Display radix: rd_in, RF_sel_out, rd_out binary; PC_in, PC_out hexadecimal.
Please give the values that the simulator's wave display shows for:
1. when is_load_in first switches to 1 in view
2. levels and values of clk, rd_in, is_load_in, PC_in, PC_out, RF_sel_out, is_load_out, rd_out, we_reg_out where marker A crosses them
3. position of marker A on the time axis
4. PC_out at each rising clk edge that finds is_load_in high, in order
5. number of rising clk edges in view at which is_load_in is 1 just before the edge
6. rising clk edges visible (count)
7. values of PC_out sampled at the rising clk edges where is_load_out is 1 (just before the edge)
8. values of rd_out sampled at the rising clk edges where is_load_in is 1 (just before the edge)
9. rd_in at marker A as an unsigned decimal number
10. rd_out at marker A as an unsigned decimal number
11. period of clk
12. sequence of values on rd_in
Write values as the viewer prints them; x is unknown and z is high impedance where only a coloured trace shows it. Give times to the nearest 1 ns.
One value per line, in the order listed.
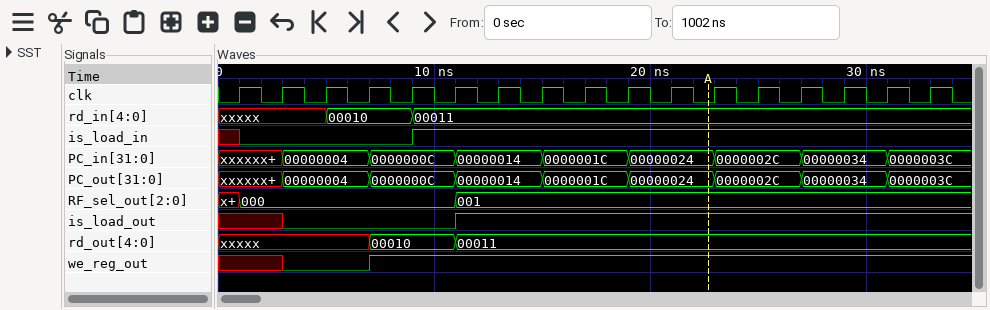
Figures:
9 ns
clk=0, rd_in=00011, is_load_in=1, PC_in=00000024, PC_out=00000024, RF_sel_out=001, is_load_out=1, rd_out=00011, we_reg_out=1
23 ns
0000000C, 00000014, 00000014, 0000001C, 0000001C, 00000024, 00000024, 0000002C, 0000002C, 00000034, 00000034, 0000003C
12
17
00000014, 00000014, 0000001C, 0000001C, 00000024, 00000024, 0000002C, 0000002C, 00000034, 00000034, 0000003C
00010, 00011, 00011, 00011, 00011, 00011, 00011, 00011, 00011, 00011, 00011, 00011
3
3
2 ns
xxxxx, 00010, 00011
